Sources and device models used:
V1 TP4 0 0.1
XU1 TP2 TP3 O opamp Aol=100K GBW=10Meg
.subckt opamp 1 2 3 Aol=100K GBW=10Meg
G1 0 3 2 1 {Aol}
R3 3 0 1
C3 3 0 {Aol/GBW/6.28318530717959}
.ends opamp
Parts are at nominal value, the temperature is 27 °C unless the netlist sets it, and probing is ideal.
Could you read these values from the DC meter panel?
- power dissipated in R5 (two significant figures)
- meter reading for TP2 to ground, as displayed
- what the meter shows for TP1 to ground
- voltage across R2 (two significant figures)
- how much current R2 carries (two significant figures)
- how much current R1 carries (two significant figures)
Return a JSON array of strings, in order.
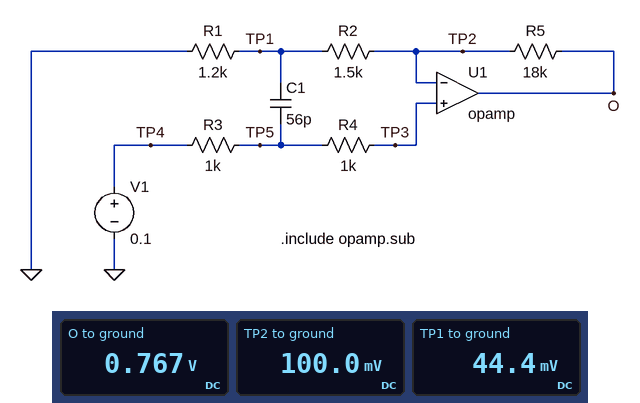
["25 µW", "100.0 mV", "44.4 mV", "56 mV", "37 µA", "37 µA"]
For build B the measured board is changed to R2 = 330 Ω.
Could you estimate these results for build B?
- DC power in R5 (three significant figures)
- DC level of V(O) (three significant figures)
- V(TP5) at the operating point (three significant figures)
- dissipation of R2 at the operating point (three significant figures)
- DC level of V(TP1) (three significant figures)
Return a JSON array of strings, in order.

["76.9 µW", "1.28 V", "100 mV", "1.41 µW", "78.4 mV"]
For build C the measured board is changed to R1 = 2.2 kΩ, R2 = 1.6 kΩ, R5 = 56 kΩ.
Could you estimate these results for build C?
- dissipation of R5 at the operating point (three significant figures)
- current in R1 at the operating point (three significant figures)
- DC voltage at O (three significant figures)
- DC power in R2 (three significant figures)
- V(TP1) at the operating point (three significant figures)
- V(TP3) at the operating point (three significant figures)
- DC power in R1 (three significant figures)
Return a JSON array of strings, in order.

["38.8 µW", "26.3 µA", "1.57 V", "1.11 µW", "57.9 mV", "100 mV", "1.52 µW"]
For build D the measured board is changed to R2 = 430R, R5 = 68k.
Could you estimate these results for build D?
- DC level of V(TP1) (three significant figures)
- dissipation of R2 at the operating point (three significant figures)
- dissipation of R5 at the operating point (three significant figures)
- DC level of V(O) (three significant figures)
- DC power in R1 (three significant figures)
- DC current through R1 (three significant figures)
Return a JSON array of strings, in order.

["73.6 mV", "1.62 µW", "256 µW", "4.27 V", "4.51 µW", "61.3 µA"]
